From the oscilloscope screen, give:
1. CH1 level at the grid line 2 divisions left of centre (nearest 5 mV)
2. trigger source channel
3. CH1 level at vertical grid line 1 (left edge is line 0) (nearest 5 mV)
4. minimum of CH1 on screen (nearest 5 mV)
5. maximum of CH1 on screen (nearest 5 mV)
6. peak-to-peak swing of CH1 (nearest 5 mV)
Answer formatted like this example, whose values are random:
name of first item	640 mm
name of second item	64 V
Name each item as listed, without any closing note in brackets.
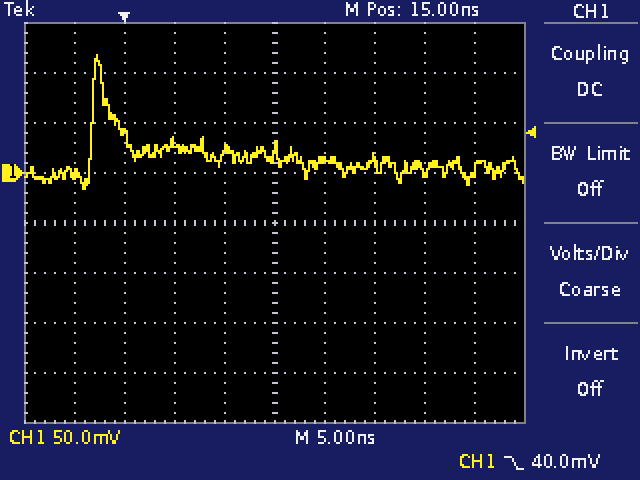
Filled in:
CH1 level at the grid line 2 divisions left of centre	30 mV
trigger source channel	CH1
CH1 level at vertical grid line 1 (left edge is line 0)	0 mV
minimum of CH1 on screen	-15 mV
maximum of CH1 on screen	120 mV
peak-to-peak swing of CH1	135 mV
